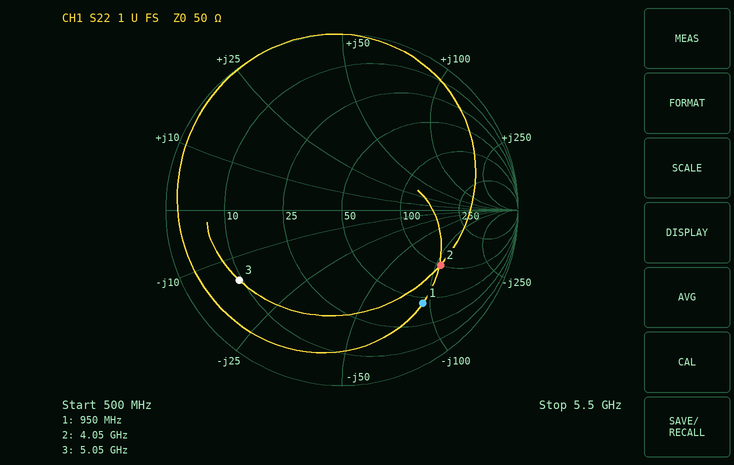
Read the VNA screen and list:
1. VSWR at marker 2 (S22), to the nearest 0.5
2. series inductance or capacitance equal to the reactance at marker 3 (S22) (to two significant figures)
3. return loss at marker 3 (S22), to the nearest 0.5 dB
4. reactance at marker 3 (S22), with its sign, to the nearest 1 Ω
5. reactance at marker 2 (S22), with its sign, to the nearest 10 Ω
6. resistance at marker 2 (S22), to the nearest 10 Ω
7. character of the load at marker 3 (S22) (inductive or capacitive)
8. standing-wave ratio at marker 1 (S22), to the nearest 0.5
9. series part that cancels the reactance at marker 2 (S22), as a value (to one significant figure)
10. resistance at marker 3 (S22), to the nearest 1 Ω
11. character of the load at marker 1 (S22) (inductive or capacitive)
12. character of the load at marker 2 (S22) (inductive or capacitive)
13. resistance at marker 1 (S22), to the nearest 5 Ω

4.5
2.1 pF
3.0 dB
-15 Ω
-110 Ω
100 Ω
capacitive
5.5
4 nH
9 Ω
capacitive
capacitive
45 Ω
